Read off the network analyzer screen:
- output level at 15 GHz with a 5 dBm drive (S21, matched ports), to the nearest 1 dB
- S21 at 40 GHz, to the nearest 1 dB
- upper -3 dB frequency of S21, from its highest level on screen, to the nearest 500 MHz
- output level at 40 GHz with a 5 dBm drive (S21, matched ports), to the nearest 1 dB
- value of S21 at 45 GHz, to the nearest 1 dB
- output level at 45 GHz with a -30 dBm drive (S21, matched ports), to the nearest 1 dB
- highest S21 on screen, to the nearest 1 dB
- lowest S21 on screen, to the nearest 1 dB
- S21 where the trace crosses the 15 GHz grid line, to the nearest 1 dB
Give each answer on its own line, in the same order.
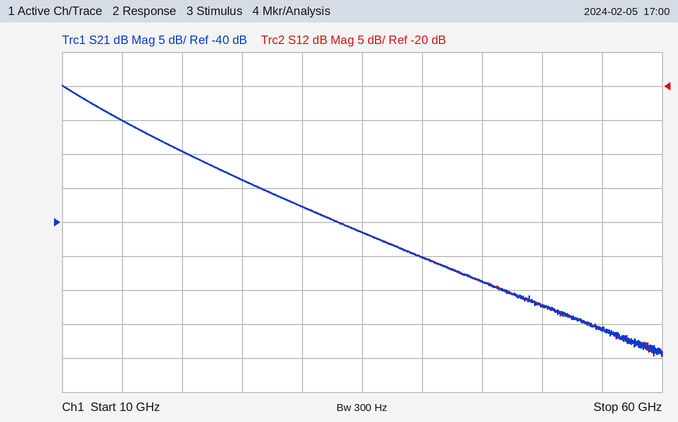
-20 dBm
-45 dB
13.0 GHz
-40 dBm
-49 dB
-79 dBm
-20 dB
-60 dB
-25 dB
